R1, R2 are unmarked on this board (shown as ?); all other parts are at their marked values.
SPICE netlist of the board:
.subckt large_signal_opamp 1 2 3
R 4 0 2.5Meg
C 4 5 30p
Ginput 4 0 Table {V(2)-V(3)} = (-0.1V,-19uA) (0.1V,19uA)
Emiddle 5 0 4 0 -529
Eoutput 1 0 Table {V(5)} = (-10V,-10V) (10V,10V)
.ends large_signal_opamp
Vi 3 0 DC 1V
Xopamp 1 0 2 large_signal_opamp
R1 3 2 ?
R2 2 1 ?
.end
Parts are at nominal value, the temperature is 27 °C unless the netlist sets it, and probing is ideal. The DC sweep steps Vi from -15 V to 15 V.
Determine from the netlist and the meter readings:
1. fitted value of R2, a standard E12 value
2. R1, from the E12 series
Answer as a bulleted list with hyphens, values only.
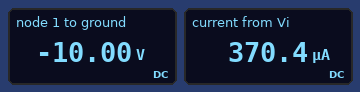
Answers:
- 27 kΩ
- 2.7 kΩ
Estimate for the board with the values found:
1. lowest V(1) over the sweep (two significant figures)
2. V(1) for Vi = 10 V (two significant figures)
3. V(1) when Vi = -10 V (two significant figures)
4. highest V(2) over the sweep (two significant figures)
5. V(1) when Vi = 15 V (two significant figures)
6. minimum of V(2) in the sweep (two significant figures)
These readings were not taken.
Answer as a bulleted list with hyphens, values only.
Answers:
- -10 V
- -10 V
- 10 V
- 13 V
- -10 V
- -13 V
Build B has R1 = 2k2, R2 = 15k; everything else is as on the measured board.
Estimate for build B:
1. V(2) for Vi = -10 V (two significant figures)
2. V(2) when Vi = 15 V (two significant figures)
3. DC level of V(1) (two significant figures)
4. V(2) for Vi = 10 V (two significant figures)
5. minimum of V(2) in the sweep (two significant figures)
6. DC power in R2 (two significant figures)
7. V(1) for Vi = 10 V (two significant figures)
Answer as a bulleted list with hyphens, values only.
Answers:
- -7.4 V
- 12 V
- -6.8 V
- 7.4 V
- -12 V
- 3.1 mW
- -10 V
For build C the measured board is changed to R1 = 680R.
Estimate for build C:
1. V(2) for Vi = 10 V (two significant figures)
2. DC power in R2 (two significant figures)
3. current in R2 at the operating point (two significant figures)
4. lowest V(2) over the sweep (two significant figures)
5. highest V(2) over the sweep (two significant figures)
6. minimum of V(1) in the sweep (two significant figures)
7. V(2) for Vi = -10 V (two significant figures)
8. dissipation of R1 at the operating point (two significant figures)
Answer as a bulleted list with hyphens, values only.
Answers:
- 9.5 V
- 4.3 mW
- 400 µA
- -14 V
- 14 V
- -10 V
- -9.5 V
- 110 µW
